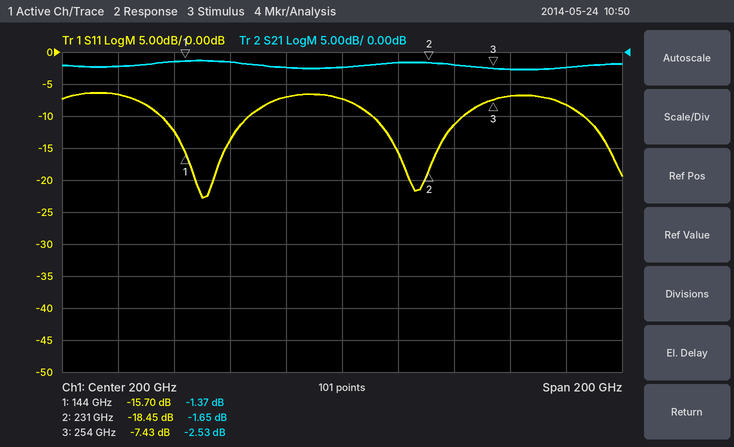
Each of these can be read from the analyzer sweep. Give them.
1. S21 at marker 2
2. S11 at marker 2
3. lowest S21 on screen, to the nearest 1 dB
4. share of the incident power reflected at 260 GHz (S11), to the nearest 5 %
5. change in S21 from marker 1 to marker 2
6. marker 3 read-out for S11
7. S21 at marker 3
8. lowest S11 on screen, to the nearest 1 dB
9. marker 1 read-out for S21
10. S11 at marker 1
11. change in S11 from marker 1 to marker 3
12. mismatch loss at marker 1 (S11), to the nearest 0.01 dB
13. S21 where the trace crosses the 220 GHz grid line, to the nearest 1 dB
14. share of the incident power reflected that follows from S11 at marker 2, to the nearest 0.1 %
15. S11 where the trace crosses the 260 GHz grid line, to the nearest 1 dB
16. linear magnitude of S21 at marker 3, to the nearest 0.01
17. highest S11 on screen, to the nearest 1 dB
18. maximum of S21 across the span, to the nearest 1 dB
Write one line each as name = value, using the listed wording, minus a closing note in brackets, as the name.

S21 at marker 2 = -1.65 dB
S11 at marker 2 = -18.45 dB
lowest S21 on screen, to the nearest 1 dB = -3 dB
share of the incident power reflected at 260 GHz (S11), to the nearest 5 % = 20 %
change in S21 from marker 1 to marker 2 = -0.28 dB
marker 3 read-out for S11 = -7.43 dB
S21 at marker 3 = -2.53 dB
lowest S11 on screen, to the nearest 1 dB = -23 dB
marker 1 read-out for S21 = -1.37 dB
S11 at marker 1 = -15.70 dB
change in S11 from marker 1 to marker 3 = 8.27 dB
mismatch loss at marker 1 (S11), to the nearest 0.01 dB = 0.12 dB
S21 where the trace crosses the 220 GHz grid line, to the nearest 1 dB = -2 dB
share of the incident power reflected that follows from S11 at marker 2, to the nearest 0.1 % = 1.4 %
S11 where the trace crosses the 260 GHz grid line, to the nearest 1 dB = -7 dB
linear magnitude of S21 at marker 3, to the nearest 0.01 = 0.75
highest S11 on screen, to the nearest 1 dB = -6 dB
maximum of S21 across the span, to the nearest 1 dB = -1 dB
